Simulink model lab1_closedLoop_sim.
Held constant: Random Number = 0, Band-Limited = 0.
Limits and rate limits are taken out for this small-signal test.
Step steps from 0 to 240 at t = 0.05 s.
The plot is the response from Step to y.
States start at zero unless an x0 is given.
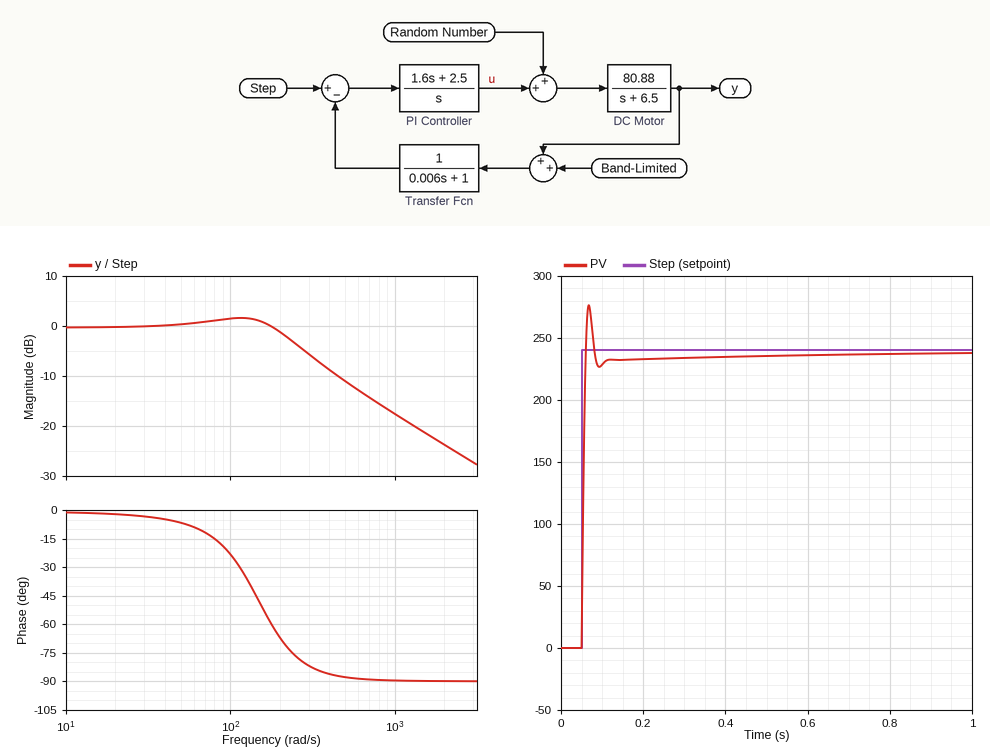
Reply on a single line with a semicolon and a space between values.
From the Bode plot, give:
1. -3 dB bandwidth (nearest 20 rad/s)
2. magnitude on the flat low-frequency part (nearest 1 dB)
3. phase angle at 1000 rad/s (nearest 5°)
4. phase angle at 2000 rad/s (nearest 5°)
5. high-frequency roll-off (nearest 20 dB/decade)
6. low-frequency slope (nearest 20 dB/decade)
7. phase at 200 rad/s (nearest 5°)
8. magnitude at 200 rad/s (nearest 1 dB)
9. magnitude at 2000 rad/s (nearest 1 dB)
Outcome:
240 rad/s; 0 dB; -90°; -90°; -20 dB/decade; 0 dB/decade; -65°; -1 dB; -24 dB
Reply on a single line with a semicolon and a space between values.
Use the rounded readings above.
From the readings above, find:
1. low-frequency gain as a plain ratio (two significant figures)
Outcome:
1.0
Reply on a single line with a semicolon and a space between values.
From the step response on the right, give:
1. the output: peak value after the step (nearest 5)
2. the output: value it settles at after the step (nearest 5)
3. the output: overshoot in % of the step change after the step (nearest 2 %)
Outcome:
275; 240; 16 %
